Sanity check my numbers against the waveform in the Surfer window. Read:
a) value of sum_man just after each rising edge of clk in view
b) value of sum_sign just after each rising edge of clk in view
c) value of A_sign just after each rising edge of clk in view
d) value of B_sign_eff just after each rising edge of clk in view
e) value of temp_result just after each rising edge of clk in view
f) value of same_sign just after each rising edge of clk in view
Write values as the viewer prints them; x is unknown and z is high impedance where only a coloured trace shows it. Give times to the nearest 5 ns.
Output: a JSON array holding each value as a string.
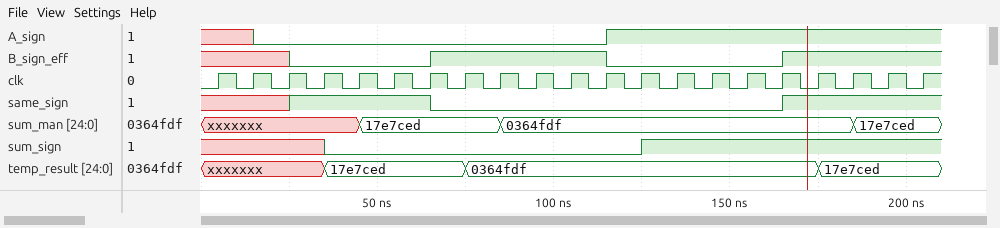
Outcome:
["xxxxxxx, xxxxxxx, xxxxxxx, xxxxxxx, 17e7ced, 17e7ced, 17e7ced, 17e7ced, 0364fdf, 0364fdf, 0364fdf, 0364fdf, 0364fdf, 0364fdf, 0364fdf, 0364fdf, 0364fdf, 0364fdf, 17e7ced, 17e7ced, 17e7ced", "x x x 0 0 0 0 0 0 0 0 0 1 1 1 1 1 1 1 1 1", "x 0 0 0 0 0 0 0 0 0 0 1 1 1 1 1 1 1 1 1 1", "x x 0 0 0 0 1 1 1 1 1 0 0 0 0 0 1 1 1 1 1", "xxxxxxx, xxxxxxx, xxxxxxx, 17e7ced, 17e7ced, 17e7ced, 17e7ced, 0364fdf, 0364fdf, 0364fdf, 0364fdf, 0364fdf, 0364fdf, 0364fdf, 0364fdf, 0364fdf, 0364fdf, 17e7ced, 17e7ced, 17e7ced, 17e7ced", "x x 1 1 1 1 0 0 0 0 0 0 0 0 0 0 1 1 1 1 1"]
